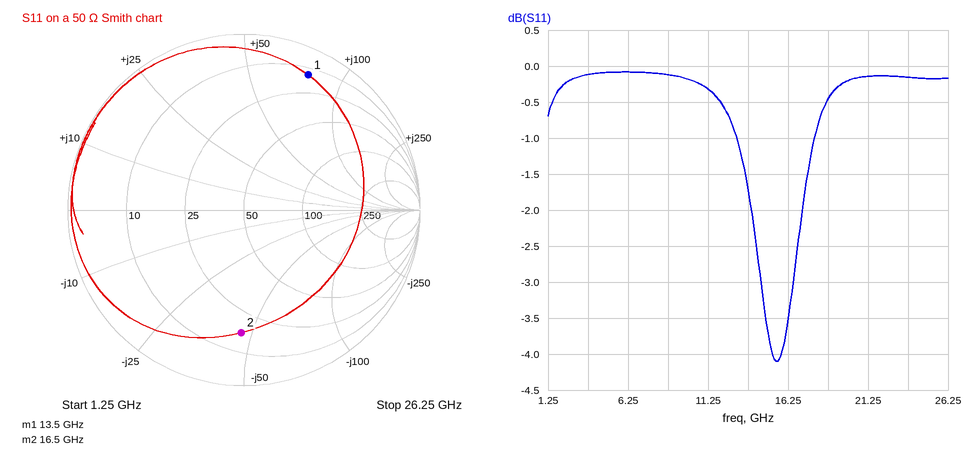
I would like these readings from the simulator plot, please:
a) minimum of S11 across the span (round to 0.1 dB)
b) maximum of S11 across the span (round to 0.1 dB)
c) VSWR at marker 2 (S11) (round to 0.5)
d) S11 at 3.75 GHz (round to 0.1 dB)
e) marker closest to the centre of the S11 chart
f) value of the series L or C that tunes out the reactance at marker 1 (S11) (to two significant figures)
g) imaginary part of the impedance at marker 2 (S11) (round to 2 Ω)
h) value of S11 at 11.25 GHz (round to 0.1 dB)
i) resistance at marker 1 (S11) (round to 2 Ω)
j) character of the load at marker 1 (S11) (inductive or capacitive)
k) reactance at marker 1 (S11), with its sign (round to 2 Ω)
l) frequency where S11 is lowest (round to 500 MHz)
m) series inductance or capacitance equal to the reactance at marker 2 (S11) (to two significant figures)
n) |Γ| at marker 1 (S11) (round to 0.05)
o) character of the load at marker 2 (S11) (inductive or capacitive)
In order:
-4.1 dB
-0.1 dB
5.5
-0.1 dB
marker 2
150 fF
-46 Ω
-0.3 dB
14 Ω
inductive
+78 Ω
15.5 GHz
210 fF
0.85
capacitive
